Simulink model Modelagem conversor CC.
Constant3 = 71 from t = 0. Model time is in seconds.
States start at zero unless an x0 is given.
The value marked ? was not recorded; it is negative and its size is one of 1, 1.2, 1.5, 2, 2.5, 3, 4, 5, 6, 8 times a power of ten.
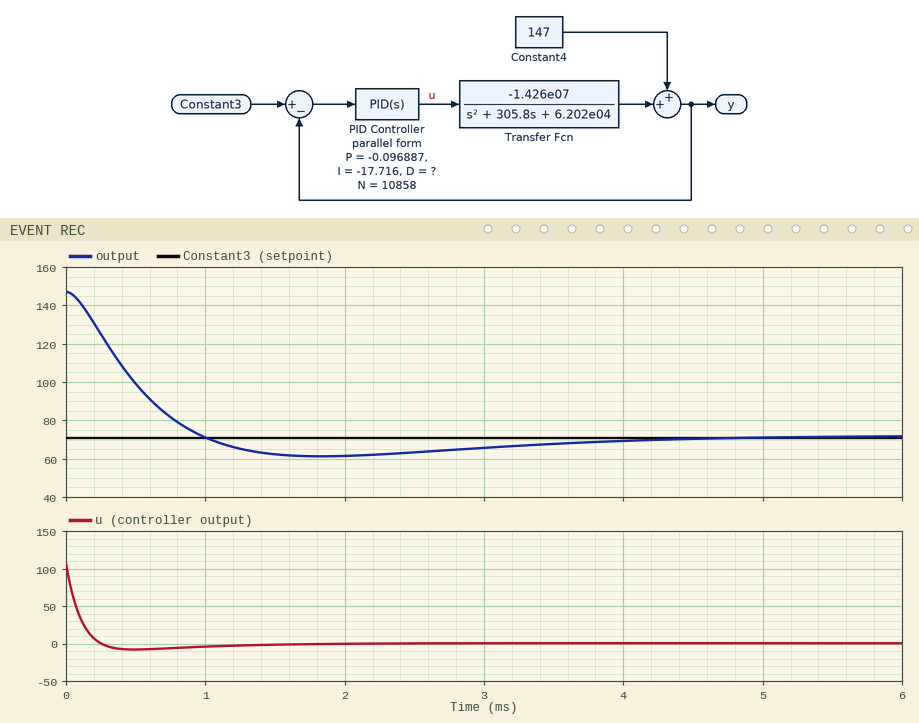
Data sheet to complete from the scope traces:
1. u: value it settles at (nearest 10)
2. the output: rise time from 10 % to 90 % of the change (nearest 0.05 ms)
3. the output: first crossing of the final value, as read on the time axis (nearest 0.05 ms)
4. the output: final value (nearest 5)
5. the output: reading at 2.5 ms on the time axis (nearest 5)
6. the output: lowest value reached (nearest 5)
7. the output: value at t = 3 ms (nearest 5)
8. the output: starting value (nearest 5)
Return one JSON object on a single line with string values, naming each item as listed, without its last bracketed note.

{"u: value it settles at": "0", "the output: rise time from 10 % to 90 % of the change": "0.70 ms", "the output: first crossing of the final value, as read on the time axis": "1.00 ms", "the output: final value": "70", "the output: reading at 2.5 ms on the time axis": "65", "the output: lowest value reached": "60", "the output: value at t = 3 ms": "65", "the output: starting value": "145"}
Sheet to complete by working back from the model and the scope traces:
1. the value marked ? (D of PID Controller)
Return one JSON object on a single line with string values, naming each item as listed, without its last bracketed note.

{"the value marked ?": "-0.00012"}
